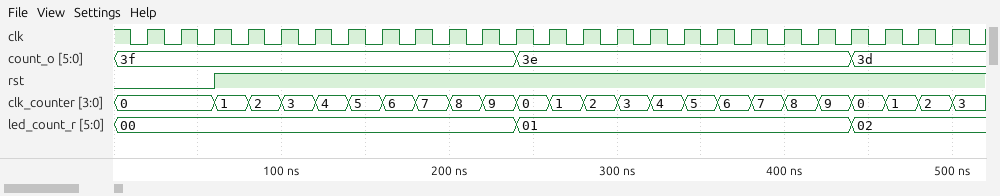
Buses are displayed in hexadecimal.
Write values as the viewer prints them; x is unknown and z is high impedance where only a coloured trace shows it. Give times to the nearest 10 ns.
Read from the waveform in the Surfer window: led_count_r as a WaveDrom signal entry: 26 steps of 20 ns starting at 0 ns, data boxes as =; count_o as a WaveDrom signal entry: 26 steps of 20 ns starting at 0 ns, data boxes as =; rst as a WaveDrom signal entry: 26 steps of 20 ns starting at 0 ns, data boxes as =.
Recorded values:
{name: 'led_count_r', wave: '=...........=.........=...', data: '00 01 02'}
{name: 'count_o', wave: '=...........=.........=...', data: '3f 3e 3d'}
{name: 'rst', wave: '0..1......................'}
